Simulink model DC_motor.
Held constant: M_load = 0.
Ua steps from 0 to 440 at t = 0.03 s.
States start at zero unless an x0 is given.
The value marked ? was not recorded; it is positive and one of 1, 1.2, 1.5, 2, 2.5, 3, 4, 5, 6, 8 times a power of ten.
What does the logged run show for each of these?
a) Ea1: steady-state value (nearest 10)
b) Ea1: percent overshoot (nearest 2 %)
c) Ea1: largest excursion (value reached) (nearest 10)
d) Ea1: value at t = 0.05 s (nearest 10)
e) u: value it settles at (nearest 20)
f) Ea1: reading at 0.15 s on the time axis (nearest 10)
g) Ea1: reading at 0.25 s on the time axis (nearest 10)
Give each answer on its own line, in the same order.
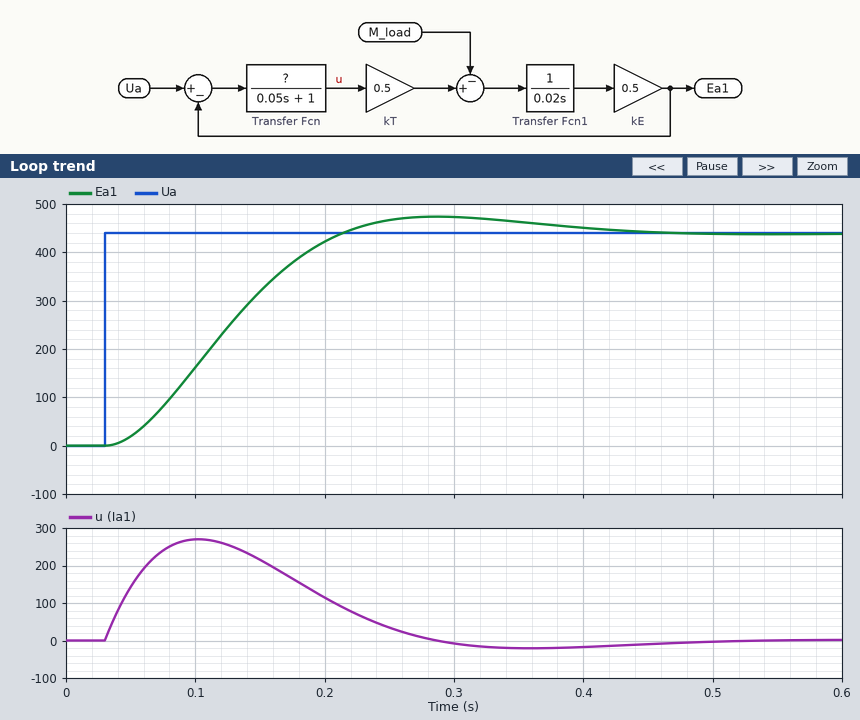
440
8 %
470
20
0
320
470
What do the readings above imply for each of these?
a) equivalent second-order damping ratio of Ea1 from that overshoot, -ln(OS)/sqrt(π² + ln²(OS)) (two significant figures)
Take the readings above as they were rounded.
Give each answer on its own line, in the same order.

0.63
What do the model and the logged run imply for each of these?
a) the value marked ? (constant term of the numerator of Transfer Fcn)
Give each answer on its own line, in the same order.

1
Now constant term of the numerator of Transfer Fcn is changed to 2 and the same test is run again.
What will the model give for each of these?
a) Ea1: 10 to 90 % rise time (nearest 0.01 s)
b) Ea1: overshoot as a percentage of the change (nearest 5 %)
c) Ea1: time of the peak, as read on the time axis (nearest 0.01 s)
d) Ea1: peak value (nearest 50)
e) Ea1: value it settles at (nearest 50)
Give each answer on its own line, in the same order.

0.07 s
20 %
0.19 s
550
450
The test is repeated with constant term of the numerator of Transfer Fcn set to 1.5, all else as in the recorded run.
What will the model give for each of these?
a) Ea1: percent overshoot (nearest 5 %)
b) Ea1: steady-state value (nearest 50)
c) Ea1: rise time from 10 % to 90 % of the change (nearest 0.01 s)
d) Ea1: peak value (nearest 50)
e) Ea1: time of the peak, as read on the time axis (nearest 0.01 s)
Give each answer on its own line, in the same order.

15 %
450
0.09 s
500
0.22 s
